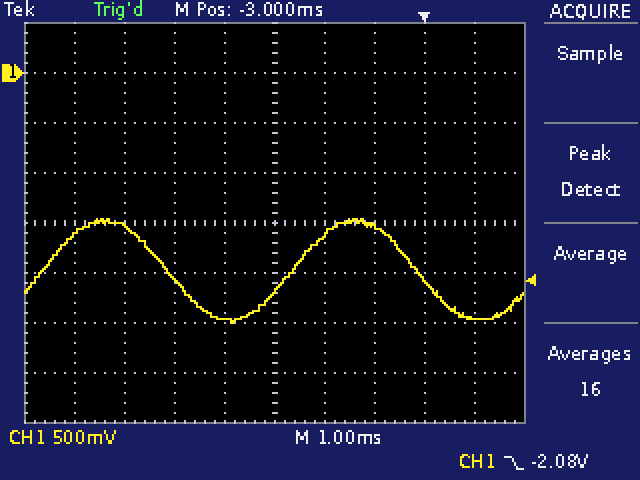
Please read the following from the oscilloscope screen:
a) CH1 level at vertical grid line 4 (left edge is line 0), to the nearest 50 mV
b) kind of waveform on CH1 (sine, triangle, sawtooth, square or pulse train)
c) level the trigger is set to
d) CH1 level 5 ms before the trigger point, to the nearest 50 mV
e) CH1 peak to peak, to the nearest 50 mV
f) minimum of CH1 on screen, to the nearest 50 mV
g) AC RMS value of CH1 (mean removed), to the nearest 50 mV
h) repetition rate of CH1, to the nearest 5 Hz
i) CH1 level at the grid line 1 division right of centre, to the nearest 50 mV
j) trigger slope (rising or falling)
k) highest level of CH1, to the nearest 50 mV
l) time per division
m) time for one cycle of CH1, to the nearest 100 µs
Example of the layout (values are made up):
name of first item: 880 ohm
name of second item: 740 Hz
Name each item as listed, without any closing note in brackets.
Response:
CH1 level at vertical grid line 4 (left edge is line 0), to the nearest 50 mV: -2.45 V
kind of waveform on CH1: sine
level the trigger is set to: -2.08 V
CH1 level 5 ms before the trigger point, to the nearest 50 mV: -2.05 V
CH1 peak to peak, to the nearest 50 mV: 1.05 V
minimum of CH1 on screen, to the nearest 50 mV: -2.50 V
AC RMS value of CH1 (mean removed), to the nearest 50 mV: 350 mV
repetition rate of CH1, to the nearest 5 Hz: 200 Hz
CH1 level at the grid line 1 division right of centre, to the nearest 50 mV: -1.60 V
trigger slope: falling
highest level of CH1, to the nearest 50 mV: -1.45 V
time per division: 1 ms
time for one cycle of CH1, to the nearest 100 µs: 5.0 ms
